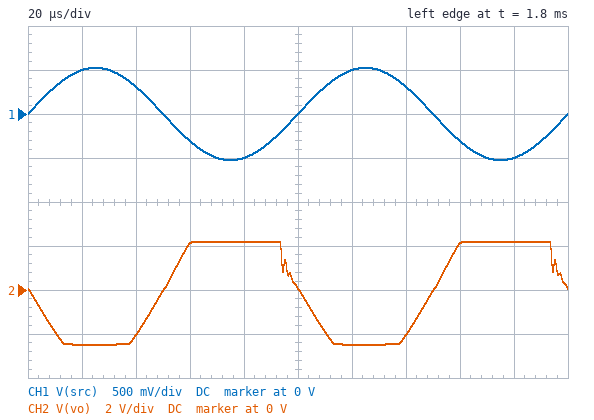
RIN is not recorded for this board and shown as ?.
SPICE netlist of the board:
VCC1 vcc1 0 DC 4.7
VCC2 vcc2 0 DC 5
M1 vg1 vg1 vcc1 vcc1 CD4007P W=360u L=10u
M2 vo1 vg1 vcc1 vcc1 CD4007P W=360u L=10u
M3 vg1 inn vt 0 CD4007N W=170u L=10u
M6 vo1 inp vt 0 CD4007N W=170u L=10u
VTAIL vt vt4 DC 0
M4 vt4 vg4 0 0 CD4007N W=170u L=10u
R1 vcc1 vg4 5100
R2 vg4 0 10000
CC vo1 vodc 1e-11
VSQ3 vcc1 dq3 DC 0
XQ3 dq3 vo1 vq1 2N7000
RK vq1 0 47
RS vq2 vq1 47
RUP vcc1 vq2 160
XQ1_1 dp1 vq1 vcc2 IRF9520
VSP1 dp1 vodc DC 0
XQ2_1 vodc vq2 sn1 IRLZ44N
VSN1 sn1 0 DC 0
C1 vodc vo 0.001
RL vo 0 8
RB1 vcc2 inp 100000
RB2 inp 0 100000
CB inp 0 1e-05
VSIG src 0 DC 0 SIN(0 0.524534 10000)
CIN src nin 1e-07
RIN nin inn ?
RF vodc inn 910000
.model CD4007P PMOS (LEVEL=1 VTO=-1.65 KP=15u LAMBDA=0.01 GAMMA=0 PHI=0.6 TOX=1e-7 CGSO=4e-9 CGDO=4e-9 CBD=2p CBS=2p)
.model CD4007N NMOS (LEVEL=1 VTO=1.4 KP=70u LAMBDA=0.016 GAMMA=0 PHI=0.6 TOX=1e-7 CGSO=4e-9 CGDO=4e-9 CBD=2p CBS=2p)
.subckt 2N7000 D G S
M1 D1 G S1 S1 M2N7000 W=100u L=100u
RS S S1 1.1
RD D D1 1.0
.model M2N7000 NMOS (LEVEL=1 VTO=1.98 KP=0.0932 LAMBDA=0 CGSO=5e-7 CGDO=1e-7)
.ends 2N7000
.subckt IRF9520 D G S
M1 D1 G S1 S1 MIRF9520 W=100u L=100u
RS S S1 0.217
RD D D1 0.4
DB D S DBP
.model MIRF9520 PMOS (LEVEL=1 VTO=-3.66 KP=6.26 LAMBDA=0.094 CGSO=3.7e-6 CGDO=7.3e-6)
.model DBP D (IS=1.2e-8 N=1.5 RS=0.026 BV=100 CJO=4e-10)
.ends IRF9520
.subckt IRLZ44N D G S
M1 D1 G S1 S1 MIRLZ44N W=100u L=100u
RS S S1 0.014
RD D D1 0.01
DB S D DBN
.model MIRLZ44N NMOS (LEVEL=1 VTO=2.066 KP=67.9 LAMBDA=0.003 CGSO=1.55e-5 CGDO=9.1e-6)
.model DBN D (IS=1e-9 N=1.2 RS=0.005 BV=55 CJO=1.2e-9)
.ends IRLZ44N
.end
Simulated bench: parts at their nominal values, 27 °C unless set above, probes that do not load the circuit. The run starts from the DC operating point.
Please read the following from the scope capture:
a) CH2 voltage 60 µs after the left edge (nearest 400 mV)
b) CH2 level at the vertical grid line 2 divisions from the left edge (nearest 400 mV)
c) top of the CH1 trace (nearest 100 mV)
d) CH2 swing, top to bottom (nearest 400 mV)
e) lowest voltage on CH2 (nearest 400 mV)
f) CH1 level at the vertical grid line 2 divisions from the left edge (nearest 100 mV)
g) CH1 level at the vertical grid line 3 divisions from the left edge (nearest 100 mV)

2.0 V
-2.0 V
500 mV
4.8 V
-2.4 V
300 mV
-300 mV
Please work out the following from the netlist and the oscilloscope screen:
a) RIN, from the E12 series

120 kΩ
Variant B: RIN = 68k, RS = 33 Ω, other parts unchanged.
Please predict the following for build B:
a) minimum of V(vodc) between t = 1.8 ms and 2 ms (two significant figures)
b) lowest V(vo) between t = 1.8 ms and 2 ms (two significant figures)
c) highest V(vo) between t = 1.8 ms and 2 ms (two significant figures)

40 mV
-2.6 V
2.1 V
